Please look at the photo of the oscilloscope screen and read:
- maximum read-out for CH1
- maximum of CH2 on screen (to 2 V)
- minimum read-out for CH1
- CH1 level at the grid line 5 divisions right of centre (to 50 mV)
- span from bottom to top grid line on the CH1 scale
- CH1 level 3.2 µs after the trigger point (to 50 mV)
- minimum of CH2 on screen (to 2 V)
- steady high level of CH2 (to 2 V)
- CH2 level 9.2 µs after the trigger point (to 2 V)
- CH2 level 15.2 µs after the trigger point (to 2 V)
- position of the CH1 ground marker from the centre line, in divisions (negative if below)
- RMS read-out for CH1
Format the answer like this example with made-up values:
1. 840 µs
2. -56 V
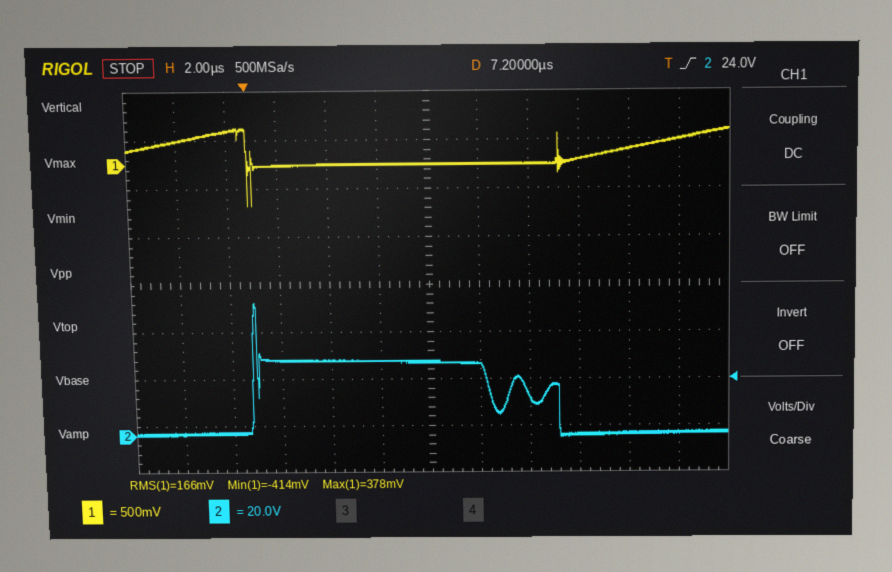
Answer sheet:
1. 378 mV
2. 56 V
3. -414 mV
4. 250 mV
5. 4 V
6. 0 mV
7. 0 V
8. 32 V
9. 30 V
10. 0 V
11. +2.5 div
12. 166 mV
